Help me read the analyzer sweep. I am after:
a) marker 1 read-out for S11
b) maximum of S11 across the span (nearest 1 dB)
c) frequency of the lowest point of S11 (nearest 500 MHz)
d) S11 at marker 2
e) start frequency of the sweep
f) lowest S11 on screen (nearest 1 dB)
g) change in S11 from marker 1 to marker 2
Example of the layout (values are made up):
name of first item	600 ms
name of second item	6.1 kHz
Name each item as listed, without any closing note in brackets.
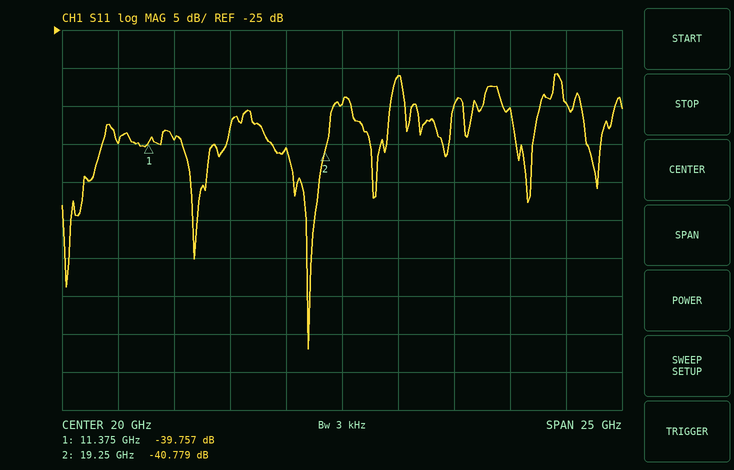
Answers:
marker 1 read-out for S11	-39.757 dB
maximum of S11 across the span	-31 dB
frequency of the lowest point of S11	18.5 GHz
S11 at marker 2	-40.779 dB
start frequency of the sweep	7.5 GHz
lowest S11 on screen	-67 dB
change in S11 from marker 1 to marker 2	-1.022 dB
